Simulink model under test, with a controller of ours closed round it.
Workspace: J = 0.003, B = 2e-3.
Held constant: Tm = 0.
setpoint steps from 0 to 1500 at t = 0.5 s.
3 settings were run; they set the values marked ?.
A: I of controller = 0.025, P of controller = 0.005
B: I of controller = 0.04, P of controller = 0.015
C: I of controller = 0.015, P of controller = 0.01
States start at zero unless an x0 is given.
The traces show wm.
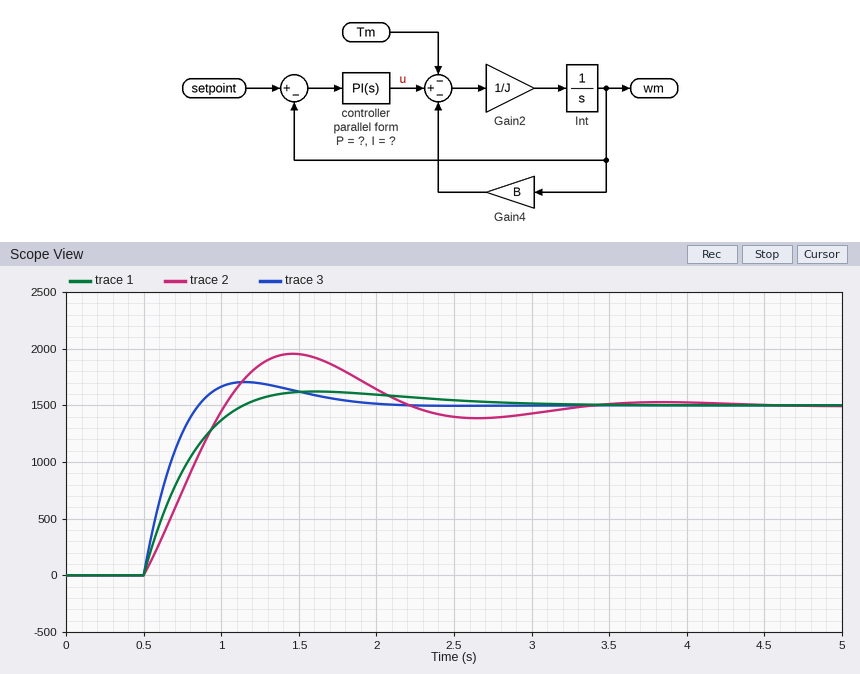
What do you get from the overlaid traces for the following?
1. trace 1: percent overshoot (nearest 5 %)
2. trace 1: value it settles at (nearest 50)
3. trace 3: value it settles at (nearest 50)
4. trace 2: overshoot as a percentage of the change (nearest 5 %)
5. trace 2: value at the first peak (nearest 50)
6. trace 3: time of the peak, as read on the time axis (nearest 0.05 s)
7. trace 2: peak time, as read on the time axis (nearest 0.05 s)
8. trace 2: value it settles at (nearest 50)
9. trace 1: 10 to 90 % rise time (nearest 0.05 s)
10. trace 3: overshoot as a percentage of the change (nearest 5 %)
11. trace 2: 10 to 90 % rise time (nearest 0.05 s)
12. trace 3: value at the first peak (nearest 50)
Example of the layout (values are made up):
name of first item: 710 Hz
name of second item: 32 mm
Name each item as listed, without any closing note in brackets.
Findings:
trace 1: percent overshoot: 10 %
trace 1: value it settles at: 1500
trace 3: value it settles at: 1500
trace 2: overshoot as a percentage of the change: 30 %
trace 2: value at the first peak: 1950
trace 3: time of the peak, as read on the time axis: 1.15 s
trace 2: peak time, as read on the time axis: 1.45 s
trace 2: value it settles at: 1500
trace 1: 10 to 90 % rise time: 0.45 s
trace 3: overshoot as a percentage of the change: 15 %
trace 2: 10 to 90 % rise time: 0.40 s
trace 3: value at the first peak: 1700
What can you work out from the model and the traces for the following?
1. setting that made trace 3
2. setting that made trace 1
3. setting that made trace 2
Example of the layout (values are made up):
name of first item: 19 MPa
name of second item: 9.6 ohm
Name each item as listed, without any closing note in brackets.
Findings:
setting that made trace 3: B
setting that made trace 1: C
setting that made trace 2: A
